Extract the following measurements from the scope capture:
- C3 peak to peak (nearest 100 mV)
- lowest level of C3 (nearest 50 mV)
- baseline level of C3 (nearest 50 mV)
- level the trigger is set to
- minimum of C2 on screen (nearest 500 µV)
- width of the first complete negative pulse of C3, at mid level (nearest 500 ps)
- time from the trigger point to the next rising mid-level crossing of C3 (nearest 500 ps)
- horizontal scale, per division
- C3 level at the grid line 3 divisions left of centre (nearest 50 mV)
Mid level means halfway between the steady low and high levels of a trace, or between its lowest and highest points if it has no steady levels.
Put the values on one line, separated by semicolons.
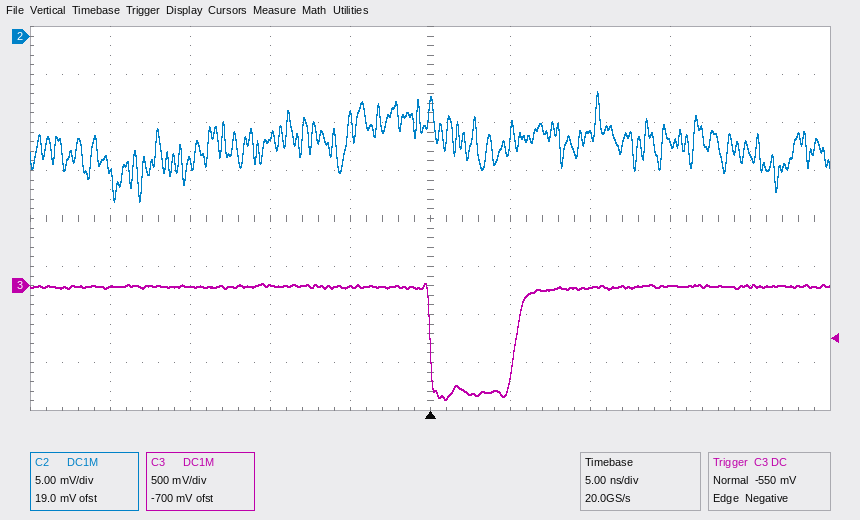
1.20 V; -1.20 V; 0 mV; -550 mV; -17.0 mV; 5.5 ns; 5.5 ns; 5 ns; 0 mV
